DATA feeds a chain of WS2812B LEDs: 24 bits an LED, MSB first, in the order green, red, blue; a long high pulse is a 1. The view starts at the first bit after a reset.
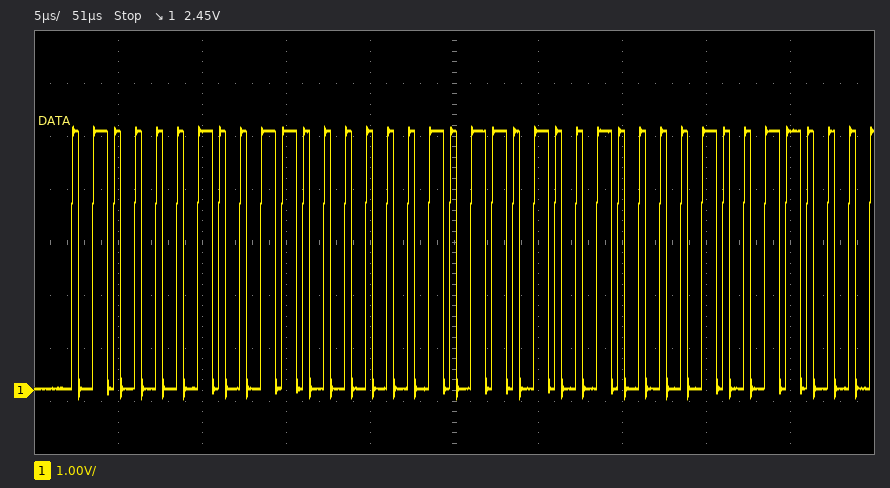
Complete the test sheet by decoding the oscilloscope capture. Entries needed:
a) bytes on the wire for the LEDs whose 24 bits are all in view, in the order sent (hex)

42 60 5A
